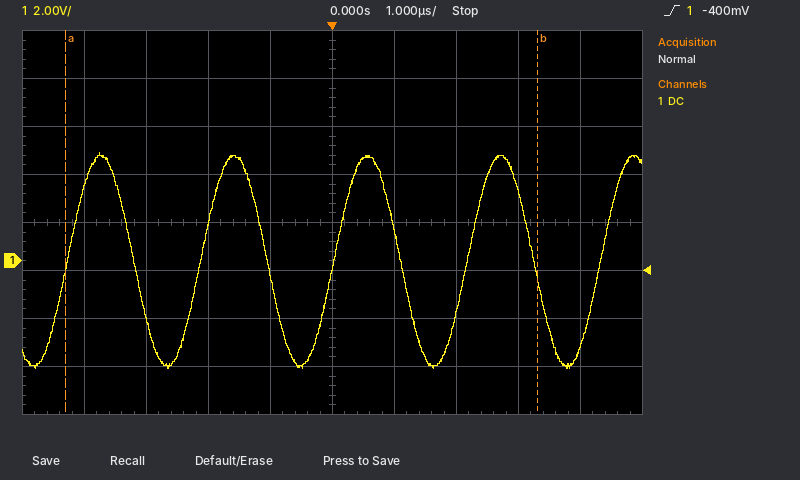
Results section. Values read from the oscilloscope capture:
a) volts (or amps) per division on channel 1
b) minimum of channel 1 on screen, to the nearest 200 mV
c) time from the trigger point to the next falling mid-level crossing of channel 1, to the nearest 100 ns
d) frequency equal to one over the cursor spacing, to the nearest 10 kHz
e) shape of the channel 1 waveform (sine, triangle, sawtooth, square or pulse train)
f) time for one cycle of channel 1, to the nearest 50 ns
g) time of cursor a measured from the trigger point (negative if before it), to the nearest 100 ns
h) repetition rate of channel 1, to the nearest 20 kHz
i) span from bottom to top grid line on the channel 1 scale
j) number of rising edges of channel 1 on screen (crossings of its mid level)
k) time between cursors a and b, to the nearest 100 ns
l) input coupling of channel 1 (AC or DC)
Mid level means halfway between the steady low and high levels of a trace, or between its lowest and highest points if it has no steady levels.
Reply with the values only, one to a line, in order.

2 V
-4.4 V
1.1 µs
130 kHz
sine
2.15 µs
-4.3 µs
460 kHz
16 V
5
7.6 µs
DC
